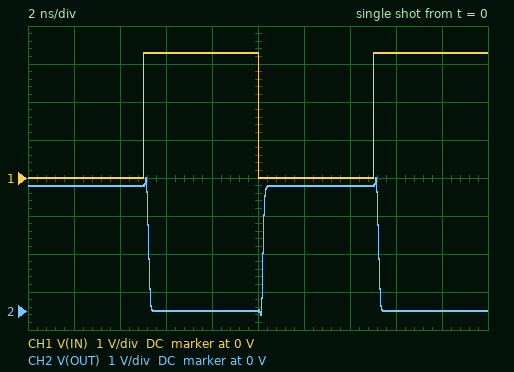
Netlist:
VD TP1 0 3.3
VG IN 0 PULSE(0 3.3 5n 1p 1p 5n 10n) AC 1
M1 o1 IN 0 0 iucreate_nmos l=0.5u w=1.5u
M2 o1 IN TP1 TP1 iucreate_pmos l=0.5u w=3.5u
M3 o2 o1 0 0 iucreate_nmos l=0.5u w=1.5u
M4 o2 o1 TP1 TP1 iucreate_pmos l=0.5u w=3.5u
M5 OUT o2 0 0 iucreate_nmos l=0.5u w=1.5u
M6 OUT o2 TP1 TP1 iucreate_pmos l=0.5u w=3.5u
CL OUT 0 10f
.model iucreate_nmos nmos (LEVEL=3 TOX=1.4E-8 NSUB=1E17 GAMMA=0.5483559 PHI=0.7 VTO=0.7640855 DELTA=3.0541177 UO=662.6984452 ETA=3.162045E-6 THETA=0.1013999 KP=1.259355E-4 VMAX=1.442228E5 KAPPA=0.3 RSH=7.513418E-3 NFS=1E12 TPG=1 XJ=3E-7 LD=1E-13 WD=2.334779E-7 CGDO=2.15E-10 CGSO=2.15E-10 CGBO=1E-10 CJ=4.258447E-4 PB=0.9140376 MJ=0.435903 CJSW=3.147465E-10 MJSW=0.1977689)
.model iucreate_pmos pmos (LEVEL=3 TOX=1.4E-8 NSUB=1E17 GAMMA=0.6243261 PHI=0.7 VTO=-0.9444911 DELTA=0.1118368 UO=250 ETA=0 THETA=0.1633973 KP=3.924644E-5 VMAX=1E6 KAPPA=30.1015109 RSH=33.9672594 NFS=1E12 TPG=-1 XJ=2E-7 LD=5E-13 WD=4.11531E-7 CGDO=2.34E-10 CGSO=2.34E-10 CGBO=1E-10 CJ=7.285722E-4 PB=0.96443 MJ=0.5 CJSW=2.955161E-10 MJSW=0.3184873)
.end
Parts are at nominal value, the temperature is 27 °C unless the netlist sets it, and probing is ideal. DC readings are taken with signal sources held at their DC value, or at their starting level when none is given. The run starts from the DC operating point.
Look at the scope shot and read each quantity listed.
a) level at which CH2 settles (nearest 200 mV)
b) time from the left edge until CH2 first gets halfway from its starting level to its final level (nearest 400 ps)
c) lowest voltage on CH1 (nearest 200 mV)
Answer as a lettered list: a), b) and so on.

a) 0 V
b) 5.2 ns
c) 0 V
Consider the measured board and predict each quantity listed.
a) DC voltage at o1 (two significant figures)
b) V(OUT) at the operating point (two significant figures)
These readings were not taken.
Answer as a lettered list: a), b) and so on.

a) 3.3 V
b) 3.3 V
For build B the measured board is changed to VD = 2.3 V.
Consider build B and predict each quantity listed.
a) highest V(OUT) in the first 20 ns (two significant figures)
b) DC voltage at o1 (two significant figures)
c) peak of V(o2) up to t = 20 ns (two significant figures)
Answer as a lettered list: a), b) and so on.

a) 2.5 V
b) 2.3 V
c) 2.6 V
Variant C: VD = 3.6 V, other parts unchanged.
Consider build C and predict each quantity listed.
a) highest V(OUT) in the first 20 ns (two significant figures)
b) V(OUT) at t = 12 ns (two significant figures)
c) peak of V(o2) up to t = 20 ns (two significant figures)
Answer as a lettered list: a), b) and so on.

a) 3.8 V
b) 3.6 V
c) 3.9 V
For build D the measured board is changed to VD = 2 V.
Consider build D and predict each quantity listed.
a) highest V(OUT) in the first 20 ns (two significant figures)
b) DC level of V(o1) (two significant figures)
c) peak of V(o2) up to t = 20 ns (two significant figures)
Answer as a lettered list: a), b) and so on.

a) 2.2 V
b) 2.0 V
c) 2.3 V
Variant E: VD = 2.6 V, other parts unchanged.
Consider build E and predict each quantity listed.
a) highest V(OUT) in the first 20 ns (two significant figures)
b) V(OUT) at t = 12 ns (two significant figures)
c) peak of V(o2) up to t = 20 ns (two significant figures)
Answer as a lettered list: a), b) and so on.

a) 2.8 V
b) 2.6 V
c) 2.9 V
